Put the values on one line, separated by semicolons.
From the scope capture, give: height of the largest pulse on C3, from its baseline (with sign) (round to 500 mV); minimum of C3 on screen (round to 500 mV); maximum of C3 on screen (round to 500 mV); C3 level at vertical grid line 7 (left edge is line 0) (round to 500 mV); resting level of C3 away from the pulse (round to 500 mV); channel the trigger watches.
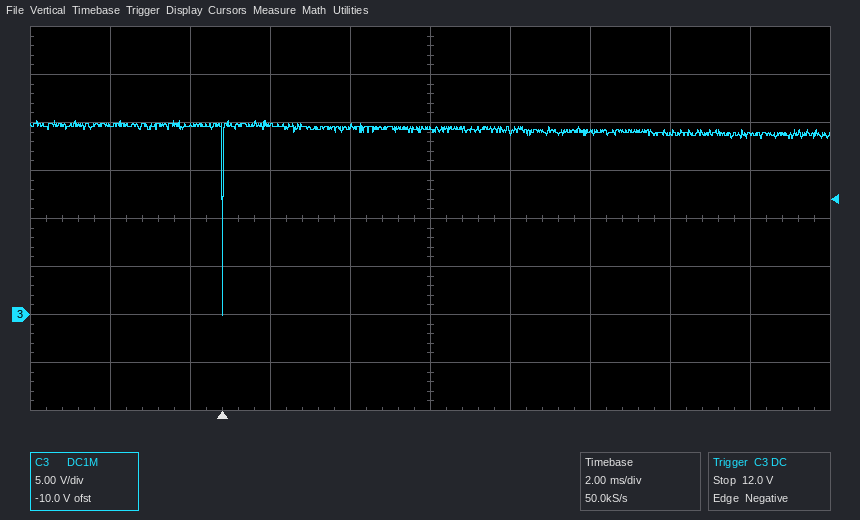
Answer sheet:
-19.5 V; 0.0 V; 20.0 V; 19.0 V; 19.5 V; C3
